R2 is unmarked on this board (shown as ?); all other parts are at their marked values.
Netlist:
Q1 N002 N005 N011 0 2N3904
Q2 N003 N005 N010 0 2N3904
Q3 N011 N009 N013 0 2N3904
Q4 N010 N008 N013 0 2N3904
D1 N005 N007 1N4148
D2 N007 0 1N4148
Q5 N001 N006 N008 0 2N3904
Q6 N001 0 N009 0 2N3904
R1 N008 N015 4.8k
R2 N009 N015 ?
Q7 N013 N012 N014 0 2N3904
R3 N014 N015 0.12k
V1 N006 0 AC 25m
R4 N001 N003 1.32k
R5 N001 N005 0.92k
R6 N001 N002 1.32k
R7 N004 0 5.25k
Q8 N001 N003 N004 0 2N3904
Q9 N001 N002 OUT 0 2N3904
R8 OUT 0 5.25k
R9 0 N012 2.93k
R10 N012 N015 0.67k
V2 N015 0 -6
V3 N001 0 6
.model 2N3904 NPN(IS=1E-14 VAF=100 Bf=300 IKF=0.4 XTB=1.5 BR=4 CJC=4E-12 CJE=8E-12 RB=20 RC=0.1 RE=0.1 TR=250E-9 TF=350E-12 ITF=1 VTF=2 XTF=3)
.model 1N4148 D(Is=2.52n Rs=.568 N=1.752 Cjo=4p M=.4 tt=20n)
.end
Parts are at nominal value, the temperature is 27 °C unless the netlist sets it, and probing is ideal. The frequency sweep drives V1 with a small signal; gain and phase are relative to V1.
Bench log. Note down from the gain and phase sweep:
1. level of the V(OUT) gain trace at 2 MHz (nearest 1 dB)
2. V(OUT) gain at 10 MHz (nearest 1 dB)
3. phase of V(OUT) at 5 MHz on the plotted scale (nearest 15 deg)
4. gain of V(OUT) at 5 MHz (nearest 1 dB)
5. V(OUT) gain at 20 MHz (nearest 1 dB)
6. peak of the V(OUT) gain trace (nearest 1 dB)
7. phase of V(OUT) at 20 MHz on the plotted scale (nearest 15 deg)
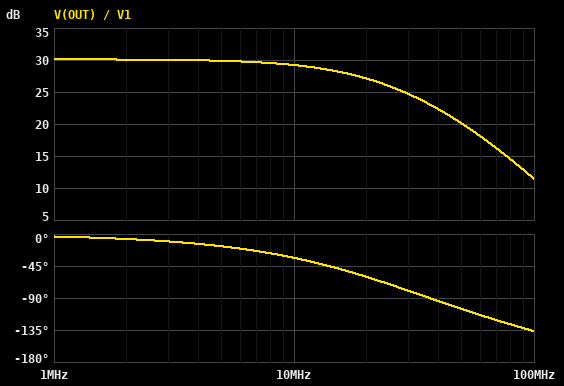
30 dB
29 dB
-15 deg
30 dB
27 dB
30 dB
-60 deg
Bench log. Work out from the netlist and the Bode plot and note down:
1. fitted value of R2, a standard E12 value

15 kΩ
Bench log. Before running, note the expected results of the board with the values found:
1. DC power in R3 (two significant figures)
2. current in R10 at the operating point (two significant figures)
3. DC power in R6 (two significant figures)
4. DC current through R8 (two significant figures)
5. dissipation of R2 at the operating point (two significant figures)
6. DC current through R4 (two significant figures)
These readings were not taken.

1.5 mW
1.7 mA
9.1 mW
360 µA
1.9 mW
870 µA
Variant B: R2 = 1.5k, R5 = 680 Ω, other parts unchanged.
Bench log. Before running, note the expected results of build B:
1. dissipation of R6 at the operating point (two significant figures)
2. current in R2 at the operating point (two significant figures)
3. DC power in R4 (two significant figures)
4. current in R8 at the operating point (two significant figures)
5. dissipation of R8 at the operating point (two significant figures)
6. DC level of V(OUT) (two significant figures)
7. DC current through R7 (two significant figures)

930 µW
3.5 mA
9.3 mW
810 µA
3.4 mW
4.2 V
360 µA
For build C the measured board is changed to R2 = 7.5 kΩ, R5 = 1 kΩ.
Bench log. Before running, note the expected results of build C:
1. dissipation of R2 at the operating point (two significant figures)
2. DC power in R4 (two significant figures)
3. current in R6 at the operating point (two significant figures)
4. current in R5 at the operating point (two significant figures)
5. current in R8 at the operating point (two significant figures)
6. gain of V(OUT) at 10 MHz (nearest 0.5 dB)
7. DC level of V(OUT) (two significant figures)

3.8 mW
2.5 mW
2.1 mA
4.7 mA
490 µA
31.5 dB
2.6 V
